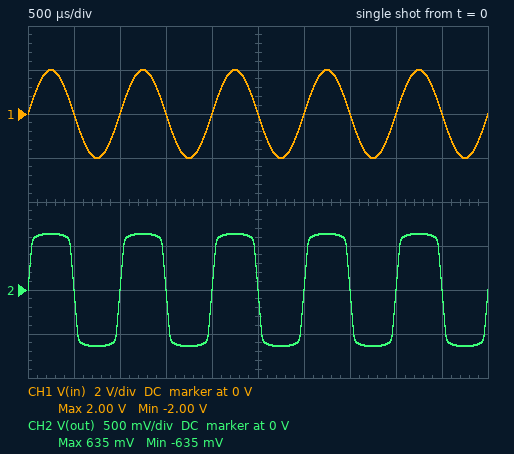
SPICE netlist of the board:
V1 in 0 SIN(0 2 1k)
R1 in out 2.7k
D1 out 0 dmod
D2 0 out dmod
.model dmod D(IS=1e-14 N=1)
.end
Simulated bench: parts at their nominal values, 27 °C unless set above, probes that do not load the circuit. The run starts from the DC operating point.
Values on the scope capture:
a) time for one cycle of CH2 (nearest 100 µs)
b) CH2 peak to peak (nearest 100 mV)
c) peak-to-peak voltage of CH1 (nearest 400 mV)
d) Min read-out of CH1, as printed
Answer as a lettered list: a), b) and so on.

a) 1.0 ms
b) 1.3 V
c) 4.0 V
d) -2.00 V
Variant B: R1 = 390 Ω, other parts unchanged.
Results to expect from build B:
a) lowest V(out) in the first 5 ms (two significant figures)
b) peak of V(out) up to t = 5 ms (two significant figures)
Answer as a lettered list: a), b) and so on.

a) -690 mV
b) 690 mV
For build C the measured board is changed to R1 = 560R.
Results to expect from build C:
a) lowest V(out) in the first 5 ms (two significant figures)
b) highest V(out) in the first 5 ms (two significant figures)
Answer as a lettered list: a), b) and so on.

a) -680 mV
b) 680 mV
